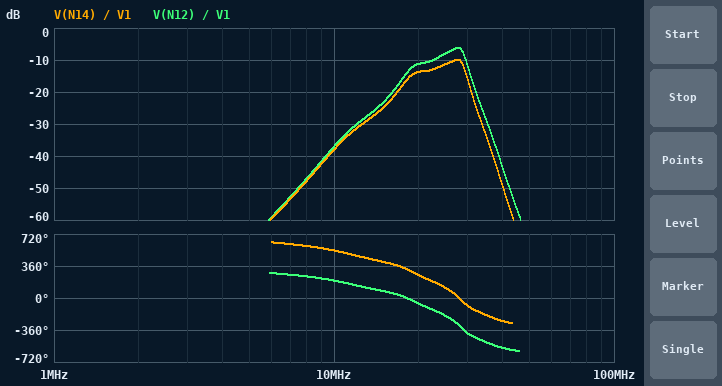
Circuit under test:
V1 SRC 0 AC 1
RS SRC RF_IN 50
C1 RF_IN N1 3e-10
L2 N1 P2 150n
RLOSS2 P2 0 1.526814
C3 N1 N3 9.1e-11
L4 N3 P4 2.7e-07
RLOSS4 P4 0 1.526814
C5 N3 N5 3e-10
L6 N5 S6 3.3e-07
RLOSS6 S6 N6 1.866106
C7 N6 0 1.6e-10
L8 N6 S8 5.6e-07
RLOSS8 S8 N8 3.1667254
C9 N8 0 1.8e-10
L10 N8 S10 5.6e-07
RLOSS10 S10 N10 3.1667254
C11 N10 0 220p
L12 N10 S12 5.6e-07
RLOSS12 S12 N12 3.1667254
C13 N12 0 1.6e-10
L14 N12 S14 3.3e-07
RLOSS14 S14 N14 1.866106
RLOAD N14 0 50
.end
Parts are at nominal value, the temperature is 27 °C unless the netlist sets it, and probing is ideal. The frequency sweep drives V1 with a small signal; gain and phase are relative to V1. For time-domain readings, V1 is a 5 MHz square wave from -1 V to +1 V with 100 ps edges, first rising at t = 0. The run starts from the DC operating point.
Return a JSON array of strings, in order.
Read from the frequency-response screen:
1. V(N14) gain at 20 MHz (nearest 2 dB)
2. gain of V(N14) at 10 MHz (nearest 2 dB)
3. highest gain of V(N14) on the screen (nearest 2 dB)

["-14 dB", "-38 dB", "-10 dB"]
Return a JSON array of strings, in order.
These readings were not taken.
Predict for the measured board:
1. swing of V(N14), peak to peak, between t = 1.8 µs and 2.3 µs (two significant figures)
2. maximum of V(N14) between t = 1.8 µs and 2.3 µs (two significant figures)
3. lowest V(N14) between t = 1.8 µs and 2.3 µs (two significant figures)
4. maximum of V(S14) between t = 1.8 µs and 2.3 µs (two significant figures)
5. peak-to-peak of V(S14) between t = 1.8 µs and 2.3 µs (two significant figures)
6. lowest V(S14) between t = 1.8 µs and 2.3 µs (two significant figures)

["190 mV", "97 mV", "-97 mV", "100 mV", "200 mV", "-100 mV"]
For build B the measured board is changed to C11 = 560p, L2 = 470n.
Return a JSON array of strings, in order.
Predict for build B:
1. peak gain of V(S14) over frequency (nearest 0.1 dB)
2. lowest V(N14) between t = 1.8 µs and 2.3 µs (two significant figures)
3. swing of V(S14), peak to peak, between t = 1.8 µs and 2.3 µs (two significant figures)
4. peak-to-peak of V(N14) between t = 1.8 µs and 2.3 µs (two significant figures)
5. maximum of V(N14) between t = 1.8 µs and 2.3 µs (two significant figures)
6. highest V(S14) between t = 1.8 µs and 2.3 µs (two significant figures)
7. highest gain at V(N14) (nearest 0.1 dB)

["-10.7 dB", "-75 mV", "160 mV", "150 mV", "75 mV", "78 mV", "-11.0 dB"]
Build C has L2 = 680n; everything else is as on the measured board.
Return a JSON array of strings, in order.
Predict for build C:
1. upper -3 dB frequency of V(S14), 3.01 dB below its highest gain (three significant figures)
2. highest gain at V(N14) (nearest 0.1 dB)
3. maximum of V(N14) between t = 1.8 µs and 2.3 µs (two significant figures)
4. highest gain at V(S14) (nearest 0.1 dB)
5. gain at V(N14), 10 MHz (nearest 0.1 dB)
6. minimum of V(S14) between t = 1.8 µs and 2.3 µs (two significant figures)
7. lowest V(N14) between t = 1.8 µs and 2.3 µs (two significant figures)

["29.8 MHz", "-9.3 dB", "160 mV", "-9.0 dB", "-20.9 dB", "-170 mV", "-160 mV"]
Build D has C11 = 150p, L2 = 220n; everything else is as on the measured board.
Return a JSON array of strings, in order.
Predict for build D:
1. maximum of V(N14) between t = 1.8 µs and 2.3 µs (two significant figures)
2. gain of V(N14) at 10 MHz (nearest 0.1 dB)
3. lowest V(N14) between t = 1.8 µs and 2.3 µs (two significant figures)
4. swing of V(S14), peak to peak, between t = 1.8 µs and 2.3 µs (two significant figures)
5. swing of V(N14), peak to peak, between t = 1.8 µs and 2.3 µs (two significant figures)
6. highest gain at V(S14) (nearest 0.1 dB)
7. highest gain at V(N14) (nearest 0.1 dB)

["150 mV", "-34.9 dB", "-150 mV", "310 mV", "300 mV", "-8.1 dB", "-8.4 dB"]
